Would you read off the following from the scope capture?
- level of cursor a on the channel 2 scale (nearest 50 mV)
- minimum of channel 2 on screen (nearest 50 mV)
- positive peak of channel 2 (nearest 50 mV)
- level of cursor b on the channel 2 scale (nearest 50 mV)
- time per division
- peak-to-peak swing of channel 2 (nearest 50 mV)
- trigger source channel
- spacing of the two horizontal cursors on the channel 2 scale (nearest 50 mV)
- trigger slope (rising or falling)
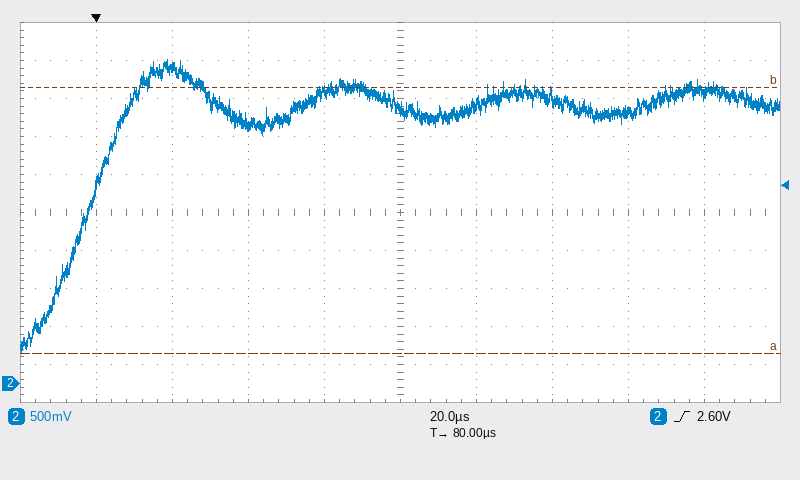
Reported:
400 mV
400 mV
4.25 V
3.90 V
20 µs
3.85 V
channel 2
3.50 V
rising
